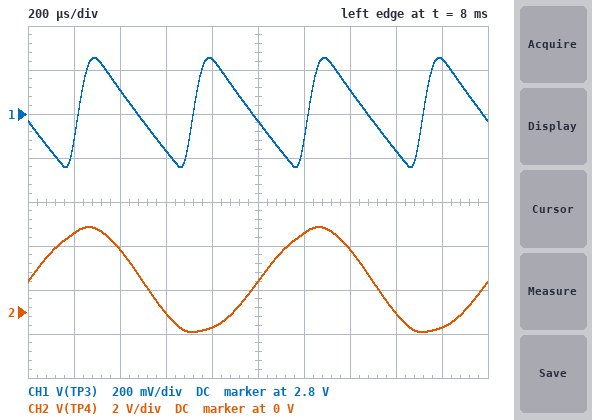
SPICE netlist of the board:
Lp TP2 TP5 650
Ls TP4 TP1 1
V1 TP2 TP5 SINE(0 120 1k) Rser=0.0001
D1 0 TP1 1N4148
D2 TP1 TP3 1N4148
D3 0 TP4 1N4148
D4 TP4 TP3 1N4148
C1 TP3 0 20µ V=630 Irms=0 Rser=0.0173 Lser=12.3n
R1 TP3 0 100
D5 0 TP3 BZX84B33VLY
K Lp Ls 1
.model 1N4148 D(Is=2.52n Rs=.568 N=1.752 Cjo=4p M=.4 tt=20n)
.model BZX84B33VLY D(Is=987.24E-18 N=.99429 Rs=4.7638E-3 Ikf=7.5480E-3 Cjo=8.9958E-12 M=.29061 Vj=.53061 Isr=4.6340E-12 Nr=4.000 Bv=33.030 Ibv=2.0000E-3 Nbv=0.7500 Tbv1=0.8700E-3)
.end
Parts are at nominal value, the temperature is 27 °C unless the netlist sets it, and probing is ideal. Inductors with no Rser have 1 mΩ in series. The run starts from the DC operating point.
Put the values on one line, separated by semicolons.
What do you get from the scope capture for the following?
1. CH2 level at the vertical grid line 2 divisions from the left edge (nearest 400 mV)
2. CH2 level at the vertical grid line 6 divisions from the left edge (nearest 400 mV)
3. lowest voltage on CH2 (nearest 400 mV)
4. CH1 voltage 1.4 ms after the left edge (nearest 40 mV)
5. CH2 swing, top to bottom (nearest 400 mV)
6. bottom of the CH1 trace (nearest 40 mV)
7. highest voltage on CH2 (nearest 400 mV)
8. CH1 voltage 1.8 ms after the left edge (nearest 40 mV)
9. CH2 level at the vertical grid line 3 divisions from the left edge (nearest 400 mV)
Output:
2.8 V; 3.6 V; -800 mV; 2.92 V; 4.8 V; 2.56 V; 4.0 V; 3.04 V; 0 V
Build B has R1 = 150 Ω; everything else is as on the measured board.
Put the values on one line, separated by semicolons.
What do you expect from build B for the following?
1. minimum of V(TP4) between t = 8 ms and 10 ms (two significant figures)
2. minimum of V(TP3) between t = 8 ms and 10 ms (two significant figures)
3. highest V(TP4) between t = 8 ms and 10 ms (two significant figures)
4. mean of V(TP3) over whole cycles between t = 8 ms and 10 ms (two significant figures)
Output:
-870 mV; 2.7 V; 3.9 V; 2.9 V
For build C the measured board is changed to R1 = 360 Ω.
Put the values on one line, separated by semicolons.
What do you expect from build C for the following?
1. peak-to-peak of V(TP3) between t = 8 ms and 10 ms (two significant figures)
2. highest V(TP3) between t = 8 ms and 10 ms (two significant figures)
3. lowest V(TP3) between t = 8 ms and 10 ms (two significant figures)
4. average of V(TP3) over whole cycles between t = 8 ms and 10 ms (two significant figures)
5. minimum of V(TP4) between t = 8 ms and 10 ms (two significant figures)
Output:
160 mV; 3.2 V; 3.0 V; 3.1 V; -810 mV
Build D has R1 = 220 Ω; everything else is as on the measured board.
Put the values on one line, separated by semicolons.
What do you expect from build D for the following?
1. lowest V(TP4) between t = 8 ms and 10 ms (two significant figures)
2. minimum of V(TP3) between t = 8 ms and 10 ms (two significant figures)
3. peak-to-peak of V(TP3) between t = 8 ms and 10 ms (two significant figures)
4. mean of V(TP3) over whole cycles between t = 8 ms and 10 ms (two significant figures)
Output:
-840 mV; 2.9 V; 250 mV; 3.0 V
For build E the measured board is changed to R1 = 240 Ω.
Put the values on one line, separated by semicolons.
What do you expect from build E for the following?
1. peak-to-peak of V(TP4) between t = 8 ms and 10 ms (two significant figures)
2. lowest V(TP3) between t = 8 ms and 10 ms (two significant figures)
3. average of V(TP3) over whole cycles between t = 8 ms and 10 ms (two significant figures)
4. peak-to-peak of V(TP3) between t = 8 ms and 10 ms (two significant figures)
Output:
4.7 V; 2.9 V; 3.0 V; 230 mV
